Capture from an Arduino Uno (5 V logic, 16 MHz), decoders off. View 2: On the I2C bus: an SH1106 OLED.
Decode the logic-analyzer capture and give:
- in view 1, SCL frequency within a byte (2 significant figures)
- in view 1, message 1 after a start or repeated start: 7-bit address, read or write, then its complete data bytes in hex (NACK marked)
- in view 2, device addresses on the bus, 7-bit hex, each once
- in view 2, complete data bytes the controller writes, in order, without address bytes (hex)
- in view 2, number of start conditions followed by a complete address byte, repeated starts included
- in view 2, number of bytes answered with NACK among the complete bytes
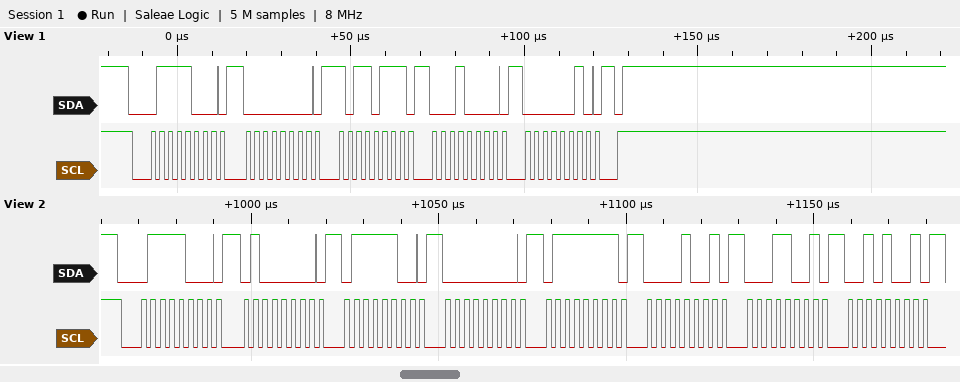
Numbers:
400 kHz
0x3C write: 00 B7 10 02
0x3C
40 7C 00 7F 09 19 29
1
0
